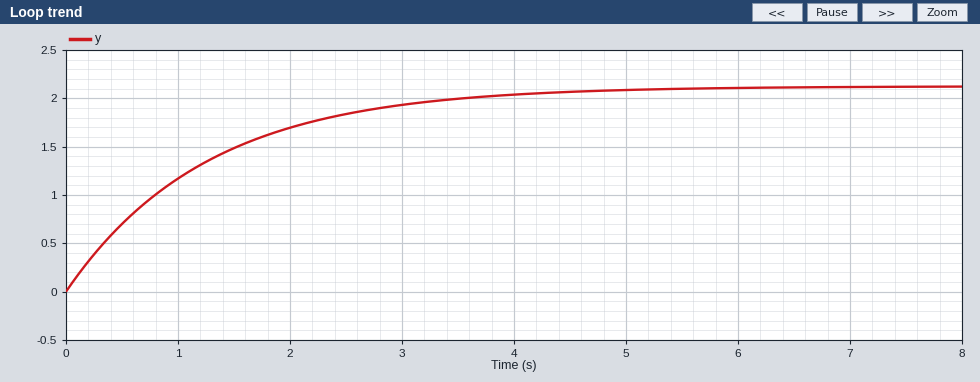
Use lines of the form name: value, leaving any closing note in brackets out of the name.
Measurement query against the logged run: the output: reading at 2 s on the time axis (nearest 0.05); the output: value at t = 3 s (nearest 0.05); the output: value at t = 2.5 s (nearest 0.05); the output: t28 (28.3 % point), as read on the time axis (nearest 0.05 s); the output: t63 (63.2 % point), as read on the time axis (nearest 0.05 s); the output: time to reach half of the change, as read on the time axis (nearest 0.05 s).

the output: reading at 2 s on the time axis: 1.70
the output: value at t = 3 s: 1.95
the output: value at t = 2.5 s: 1.85
the output: t28 (28.3 % point), as read on the time axis: 0.40 s
the output: t63 (63.2 % point), as read on the time axis: 1.25 s
the output: time to reach half of the change, as read on the time axis: 0.85 s
